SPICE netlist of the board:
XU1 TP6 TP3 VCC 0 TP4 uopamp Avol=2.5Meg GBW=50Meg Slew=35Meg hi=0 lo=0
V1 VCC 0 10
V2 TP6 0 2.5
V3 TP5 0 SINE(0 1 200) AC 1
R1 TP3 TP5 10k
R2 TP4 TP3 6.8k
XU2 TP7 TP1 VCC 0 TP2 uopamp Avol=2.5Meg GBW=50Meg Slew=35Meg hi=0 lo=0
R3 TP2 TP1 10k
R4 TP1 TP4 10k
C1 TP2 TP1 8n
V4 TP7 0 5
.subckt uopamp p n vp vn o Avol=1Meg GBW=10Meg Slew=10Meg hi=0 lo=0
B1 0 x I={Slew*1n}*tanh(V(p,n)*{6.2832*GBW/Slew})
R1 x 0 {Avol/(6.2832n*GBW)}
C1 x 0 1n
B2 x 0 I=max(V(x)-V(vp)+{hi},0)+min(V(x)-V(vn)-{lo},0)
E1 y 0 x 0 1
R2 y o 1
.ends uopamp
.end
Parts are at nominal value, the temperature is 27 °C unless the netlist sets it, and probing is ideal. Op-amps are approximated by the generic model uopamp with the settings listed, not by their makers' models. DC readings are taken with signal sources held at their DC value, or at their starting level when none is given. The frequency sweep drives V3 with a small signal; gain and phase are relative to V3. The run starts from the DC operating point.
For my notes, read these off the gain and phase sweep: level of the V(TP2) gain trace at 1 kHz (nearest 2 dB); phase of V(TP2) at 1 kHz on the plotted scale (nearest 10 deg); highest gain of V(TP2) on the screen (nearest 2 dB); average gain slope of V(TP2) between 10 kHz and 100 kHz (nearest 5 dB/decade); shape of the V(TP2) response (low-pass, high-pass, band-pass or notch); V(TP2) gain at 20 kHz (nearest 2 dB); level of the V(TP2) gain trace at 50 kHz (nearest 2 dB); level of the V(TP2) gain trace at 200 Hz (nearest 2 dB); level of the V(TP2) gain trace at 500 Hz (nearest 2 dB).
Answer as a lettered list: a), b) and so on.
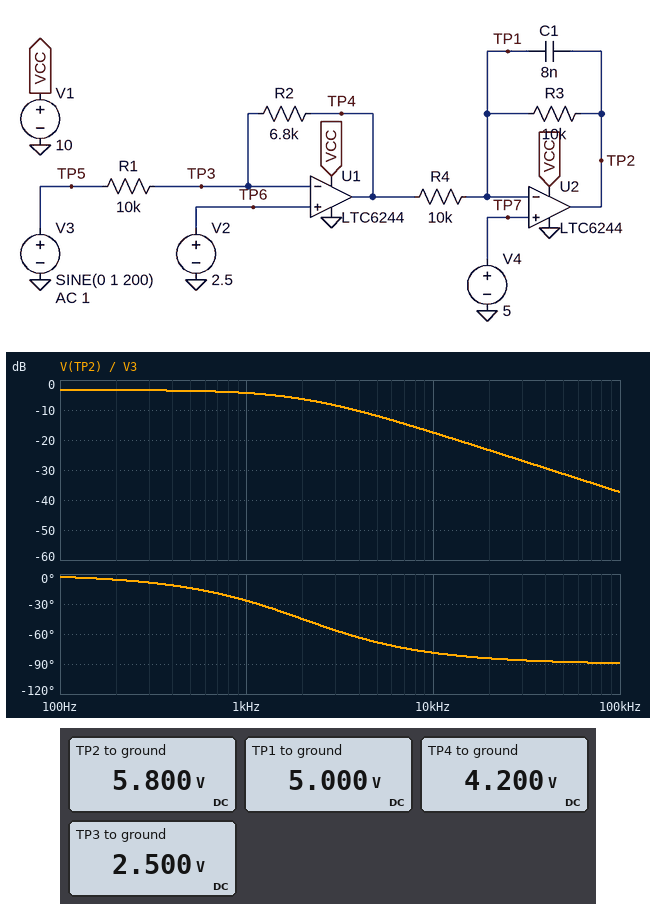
a) -4 dB
b) -30 deg
c) -4 dB
d) -20 dB/decade
e) low-pass
f) -24 dB
g) -32 dB
h) -4 dB
i) -4 dB
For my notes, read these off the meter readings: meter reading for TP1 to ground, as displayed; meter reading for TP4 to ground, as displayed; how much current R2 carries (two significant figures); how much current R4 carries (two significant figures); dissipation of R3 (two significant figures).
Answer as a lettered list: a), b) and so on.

a) 5.000 V
b) 4.200 V
c) 250 µA
d) 80 µA
e) 64 µW
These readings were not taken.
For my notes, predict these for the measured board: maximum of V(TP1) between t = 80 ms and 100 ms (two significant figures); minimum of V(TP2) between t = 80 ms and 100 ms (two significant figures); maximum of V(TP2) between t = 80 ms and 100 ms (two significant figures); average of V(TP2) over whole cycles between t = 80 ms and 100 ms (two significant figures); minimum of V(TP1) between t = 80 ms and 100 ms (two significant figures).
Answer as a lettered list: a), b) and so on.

a) 5.0 V
b) 5.1 V
c) 6.5 V
d) 5.8 V
e) 5.0 V
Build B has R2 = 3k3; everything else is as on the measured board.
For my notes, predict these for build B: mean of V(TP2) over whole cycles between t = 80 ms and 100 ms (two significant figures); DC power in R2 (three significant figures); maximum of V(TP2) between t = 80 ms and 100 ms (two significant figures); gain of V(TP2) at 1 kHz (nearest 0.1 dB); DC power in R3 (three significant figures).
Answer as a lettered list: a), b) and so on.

a) 6.7 V
b) 206 µW
c) 7.0 V
d) -10.6 dB
e) 281 µW
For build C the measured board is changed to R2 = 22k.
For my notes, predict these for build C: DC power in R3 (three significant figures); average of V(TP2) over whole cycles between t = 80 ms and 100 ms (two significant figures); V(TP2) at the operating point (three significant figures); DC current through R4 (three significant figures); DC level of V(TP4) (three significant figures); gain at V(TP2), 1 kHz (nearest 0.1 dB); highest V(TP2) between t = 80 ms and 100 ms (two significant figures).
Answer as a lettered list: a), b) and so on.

a) 900 µW
b) 2.0 V
c) 2.00 V
d) 300 µA
e) 8.00 V
f) 5.9 dB
g) 4.2 V
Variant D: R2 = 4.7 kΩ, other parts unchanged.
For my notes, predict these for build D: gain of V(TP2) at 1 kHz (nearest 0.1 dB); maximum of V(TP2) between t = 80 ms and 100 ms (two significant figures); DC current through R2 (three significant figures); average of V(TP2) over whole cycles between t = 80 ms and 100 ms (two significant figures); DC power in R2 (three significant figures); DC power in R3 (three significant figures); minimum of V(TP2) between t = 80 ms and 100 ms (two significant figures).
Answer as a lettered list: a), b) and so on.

a) -7.5 dB
b) 6.8 V
c) 250 µA
d) 6.3 V
e) 294 µW
f) 176 µW
g) 5.9 V
